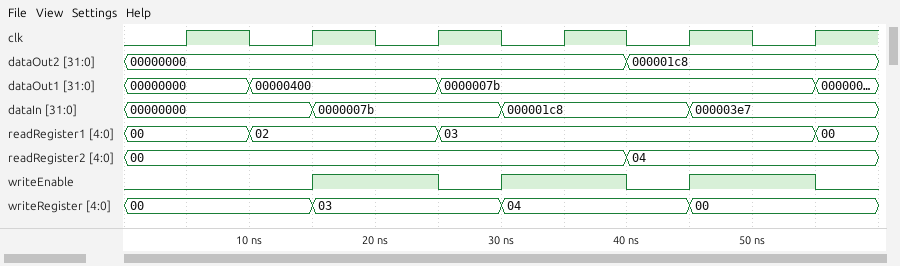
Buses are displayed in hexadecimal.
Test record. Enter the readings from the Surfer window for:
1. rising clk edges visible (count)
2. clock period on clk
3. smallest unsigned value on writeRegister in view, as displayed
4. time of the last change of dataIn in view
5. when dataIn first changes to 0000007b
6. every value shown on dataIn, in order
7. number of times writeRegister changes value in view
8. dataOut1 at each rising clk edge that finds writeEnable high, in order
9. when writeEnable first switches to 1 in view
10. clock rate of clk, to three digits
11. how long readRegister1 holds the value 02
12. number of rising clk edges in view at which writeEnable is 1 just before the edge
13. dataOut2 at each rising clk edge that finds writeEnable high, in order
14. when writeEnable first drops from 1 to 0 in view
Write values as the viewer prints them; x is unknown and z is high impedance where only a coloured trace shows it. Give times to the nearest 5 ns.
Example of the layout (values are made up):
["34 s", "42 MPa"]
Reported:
["6", "10 ns", "00", "45 ns", "15 ns", "00000000, 0000007b, 000001c8, 000003e7", "3", "00000400, 0000007b, 0000007b", "15 ns", "100 MHz", "15 ns", "3", "00000000, 00000000, 000001c8", "25 ns"]
